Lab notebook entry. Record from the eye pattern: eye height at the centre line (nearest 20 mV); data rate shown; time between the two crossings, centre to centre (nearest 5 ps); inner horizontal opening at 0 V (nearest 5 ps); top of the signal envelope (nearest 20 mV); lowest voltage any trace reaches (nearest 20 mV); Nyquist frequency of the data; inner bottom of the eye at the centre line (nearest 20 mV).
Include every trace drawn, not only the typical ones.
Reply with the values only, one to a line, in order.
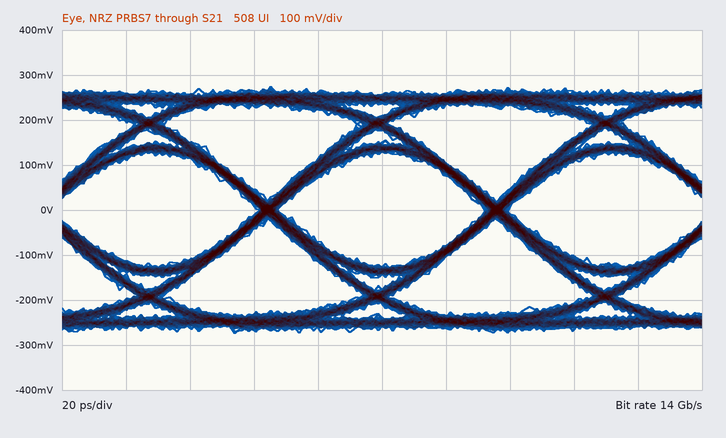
260 mV
14 Gb/s
70 ps
65 ps
280 mV
-280 mV
7 GHz
-120 mV
